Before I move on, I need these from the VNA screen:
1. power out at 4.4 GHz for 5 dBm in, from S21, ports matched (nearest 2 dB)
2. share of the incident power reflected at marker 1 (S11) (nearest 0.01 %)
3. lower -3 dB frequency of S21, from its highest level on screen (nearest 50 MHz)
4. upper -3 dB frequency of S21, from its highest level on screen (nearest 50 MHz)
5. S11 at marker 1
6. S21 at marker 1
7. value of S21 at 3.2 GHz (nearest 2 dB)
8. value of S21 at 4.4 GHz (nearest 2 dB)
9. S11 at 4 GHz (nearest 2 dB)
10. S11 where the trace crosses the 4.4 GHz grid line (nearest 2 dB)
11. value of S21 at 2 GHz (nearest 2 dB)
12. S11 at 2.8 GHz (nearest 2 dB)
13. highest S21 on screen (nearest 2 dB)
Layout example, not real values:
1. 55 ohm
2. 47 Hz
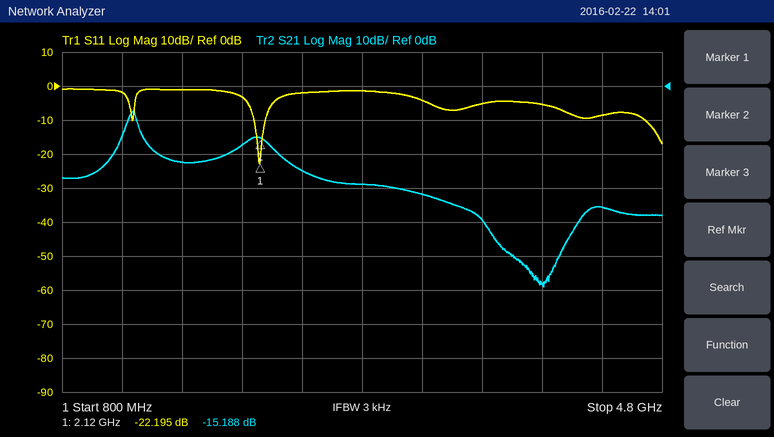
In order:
1. -30 dBm
2. 0.60 %
3. 1.25 GHz
4. 1.30 GHz
5. -22.195 dB
6. -15.188 dB
7. -32 dB
8. -36 dB
9. -6 dB
10. -8 dB
11. -18 dB
12. -2 dB
13. -8 dB
